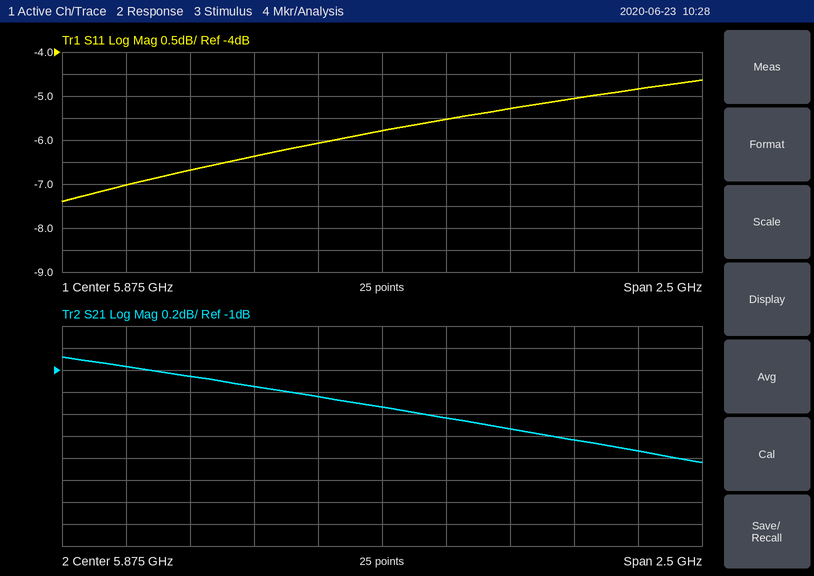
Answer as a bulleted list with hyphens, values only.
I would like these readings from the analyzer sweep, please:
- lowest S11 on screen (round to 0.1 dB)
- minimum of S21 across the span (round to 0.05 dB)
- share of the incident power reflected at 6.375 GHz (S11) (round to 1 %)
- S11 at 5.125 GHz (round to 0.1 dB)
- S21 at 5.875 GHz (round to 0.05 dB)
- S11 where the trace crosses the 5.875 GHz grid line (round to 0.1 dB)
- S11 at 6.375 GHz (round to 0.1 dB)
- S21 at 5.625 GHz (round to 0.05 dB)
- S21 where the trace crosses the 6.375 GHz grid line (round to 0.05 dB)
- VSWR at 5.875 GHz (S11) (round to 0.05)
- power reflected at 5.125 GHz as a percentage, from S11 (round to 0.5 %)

- -7.4 dB
- -1.85 dB
- 30 %
- -6.7 dB
- -1.35 dB
- -5.8 dB
- -5.3 dB
- -1.25 dB
- -1.55 dB
- 3.10
- 21.5 %
